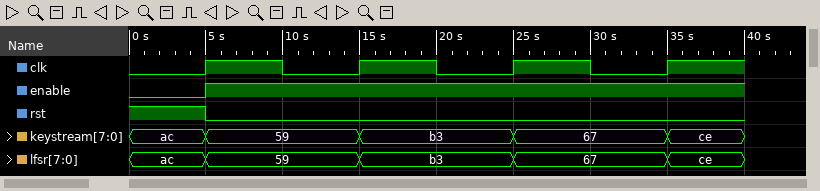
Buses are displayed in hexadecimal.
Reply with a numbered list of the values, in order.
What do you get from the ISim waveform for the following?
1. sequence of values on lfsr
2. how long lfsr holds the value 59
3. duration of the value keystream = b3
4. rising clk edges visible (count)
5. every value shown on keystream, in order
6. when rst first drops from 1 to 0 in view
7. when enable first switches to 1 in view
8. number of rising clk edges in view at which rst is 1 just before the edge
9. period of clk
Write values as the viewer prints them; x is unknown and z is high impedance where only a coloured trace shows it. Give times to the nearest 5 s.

1. ac, 59, b3, 67, ce
2. 10 s
3. 10 s
4. 4
5. ac, 59, b3, 67, ce
6. 5 s
7. 5 s
8. 1
9. 10 s
